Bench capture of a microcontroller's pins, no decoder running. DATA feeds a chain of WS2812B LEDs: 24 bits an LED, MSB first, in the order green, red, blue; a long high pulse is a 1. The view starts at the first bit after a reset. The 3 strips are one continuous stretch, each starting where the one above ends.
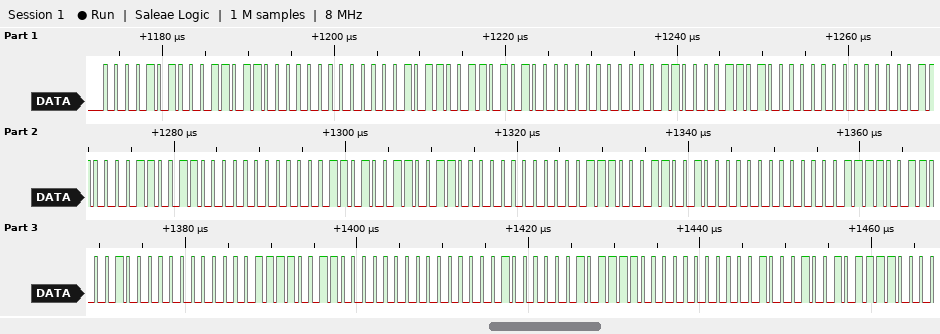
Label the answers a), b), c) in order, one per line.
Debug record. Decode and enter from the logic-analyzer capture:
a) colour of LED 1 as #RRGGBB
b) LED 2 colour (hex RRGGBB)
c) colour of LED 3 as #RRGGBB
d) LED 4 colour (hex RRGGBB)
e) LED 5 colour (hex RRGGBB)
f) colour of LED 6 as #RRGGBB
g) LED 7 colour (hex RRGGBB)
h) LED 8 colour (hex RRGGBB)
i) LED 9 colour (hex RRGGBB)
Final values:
a) #360A00
b) #350B00
c) #340C00
d) #330C00
e) #330D00
f) #320E00
g) #310F00
h) #300F00
i) #2F1000
